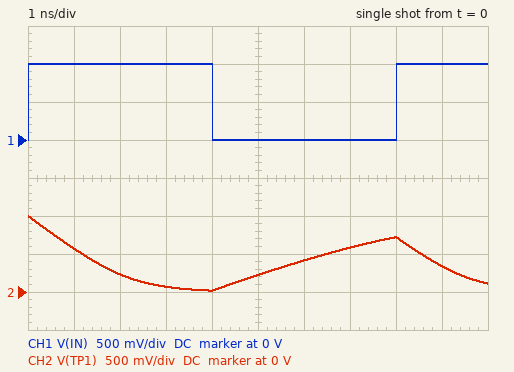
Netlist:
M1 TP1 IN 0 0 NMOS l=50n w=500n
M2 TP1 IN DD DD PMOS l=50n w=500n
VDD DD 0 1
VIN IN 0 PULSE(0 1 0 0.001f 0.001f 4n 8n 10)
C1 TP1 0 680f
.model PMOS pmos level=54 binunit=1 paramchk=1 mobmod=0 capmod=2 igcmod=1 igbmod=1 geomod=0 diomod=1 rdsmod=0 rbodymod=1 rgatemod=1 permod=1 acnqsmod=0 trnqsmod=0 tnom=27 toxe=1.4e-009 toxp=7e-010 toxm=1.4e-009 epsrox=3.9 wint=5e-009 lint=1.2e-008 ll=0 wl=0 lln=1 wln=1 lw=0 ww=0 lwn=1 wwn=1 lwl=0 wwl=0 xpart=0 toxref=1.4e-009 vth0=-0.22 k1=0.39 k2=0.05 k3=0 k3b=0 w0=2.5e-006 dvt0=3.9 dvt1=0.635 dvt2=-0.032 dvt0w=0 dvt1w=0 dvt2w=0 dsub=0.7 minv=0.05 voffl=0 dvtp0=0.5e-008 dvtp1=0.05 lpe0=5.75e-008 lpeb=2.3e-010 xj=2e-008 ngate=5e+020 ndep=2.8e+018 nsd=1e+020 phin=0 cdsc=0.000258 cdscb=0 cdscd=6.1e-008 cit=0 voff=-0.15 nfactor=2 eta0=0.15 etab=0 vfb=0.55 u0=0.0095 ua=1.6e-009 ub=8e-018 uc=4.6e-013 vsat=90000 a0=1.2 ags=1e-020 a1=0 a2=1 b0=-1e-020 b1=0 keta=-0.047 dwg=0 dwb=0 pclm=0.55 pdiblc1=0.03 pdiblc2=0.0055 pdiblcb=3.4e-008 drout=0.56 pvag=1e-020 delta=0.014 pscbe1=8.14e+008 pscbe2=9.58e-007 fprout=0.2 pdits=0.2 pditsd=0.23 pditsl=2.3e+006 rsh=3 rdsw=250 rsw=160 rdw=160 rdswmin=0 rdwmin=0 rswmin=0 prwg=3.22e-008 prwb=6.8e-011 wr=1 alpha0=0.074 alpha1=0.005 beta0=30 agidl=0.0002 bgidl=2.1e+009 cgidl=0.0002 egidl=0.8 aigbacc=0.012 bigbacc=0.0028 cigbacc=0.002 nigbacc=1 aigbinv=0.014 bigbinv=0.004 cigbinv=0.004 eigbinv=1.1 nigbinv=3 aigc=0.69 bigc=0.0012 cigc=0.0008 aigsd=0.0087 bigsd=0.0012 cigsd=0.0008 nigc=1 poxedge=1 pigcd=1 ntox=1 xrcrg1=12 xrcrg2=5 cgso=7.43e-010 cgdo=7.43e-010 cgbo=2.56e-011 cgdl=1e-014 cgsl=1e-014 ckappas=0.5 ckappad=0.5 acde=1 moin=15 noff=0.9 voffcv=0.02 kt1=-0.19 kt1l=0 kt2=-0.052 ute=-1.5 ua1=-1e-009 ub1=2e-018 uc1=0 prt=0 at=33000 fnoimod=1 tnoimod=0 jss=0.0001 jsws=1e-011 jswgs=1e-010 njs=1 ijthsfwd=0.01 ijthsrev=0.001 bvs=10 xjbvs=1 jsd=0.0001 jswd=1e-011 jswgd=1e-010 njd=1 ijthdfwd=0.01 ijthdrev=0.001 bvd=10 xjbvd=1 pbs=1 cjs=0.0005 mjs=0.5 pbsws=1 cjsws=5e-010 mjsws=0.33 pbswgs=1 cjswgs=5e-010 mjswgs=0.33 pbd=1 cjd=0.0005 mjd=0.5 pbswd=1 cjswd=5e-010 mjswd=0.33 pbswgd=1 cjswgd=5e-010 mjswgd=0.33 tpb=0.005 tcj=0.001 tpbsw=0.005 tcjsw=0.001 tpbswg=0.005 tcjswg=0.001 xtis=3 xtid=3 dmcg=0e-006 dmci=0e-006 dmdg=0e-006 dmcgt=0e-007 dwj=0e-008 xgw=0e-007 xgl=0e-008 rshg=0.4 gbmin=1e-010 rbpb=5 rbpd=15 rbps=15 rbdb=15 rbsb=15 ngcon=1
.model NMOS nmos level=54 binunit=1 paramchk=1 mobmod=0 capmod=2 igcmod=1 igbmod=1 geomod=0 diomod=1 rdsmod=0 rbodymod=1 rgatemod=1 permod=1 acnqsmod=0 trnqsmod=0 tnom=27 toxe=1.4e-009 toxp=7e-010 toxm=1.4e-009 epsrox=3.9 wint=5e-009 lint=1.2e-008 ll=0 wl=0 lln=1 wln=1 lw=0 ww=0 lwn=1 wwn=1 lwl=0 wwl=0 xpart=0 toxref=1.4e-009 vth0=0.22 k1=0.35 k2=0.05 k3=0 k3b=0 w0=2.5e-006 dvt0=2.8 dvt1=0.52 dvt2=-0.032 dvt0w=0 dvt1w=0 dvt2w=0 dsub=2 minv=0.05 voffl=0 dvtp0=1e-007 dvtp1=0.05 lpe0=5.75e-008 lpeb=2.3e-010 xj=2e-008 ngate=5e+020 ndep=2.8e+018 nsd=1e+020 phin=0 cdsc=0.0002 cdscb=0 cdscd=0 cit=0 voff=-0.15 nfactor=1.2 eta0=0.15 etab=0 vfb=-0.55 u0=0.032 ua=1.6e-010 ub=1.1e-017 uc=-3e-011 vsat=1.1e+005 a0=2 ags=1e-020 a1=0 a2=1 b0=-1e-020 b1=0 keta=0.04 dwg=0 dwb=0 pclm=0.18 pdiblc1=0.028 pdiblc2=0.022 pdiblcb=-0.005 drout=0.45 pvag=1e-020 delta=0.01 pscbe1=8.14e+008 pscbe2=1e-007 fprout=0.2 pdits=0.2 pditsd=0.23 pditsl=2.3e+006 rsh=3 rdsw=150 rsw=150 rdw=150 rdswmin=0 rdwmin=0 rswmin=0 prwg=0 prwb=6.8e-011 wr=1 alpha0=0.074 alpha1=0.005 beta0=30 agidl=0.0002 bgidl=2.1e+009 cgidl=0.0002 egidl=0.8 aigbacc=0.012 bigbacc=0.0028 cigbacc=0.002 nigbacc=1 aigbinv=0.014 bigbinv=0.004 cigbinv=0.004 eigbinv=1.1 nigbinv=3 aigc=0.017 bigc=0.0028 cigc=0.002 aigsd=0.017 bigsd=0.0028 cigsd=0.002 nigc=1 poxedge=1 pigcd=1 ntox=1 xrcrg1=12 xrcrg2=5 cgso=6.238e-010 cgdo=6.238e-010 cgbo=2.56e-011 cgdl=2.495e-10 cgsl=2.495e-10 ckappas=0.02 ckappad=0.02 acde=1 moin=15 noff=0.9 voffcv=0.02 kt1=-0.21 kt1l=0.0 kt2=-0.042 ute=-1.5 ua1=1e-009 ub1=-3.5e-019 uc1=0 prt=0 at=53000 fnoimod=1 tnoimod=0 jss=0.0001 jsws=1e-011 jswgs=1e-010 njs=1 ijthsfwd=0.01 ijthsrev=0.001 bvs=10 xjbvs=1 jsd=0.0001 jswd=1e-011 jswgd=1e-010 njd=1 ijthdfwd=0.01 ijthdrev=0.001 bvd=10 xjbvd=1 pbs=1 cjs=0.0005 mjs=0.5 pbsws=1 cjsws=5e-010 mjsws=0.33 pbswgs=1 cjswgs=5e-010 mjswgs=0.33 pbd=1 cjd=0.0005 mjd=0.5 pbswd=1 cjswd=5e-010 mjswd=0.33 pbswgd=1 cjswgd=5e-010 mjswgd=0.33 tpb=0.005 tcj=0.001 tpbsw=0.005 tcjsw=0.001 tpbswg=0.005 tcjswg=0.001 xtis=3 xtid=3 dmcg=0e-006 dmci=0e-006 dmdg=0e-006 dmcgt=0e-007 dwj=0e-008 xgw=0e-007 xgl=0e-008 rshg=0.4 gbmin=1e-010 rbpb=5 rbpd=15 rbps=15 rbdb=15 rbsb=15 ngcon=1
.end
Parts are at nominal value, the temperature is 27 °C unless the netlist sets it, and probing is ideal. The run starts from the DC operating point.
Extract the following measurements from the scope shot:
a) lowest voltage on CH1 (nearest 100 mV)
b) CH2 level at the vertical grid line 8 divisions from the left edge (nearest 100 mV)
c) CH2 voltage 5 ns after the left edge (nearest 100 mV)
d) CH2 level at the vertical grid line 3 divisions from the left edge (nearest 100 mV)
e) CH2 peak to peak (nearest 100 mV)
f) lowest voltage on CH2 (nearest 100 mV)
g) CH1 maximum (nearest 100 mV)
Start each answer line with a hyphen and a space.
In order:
- 0 V
- 700 mV
- 200 mV
- 100 mV
- 1.0 V
- 0 V
- 1.0 V
